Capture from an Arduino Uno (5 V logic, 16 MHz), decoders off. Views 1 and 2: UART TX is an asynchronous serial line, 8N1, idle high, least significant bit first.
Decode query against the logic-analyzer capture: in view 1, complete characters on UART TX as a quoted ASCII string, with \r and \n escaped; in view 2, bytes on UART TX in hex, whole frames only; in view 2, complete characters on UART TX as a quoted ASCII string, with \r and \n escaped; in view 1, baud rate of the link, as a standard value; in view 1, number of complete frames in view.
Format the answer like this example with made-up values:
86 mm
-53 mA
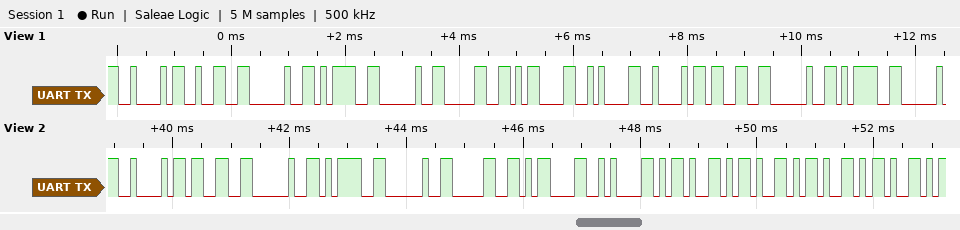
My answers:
"B2 = 0\r\nB3 ="
42 33 20 3D 20 30 0D 0A 2D 2D 2D 2D
"B3 = 0\r\n----"
9600 baud
12
